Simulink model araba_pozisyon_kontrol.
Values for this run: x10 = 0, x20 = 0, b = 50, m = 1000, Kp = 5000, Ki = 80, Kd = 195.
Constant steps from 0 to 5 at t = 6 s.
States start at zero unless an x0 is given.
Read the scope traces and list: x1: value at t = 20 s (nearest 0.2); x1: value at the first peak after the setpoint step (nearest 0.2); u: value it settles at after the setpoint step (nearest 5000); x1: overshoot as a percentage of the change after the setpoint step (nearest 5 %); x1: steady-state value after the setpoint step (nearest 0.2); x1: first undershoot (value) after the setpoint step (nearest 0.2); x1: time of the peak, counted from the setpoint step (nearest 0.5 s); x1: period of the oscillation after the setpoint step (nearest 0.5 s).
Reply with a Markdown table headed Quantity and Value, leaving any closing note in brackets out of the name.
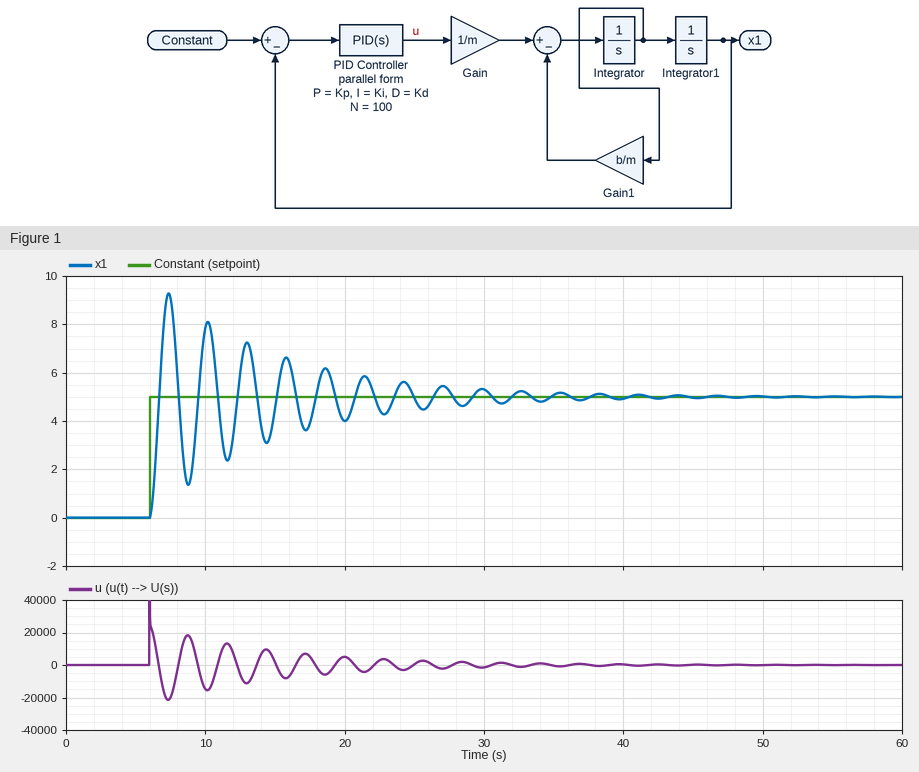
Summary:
| Quantity | Value |
|---|---|
| x1: value at t = 20 s | 4.0 |
| x1: value at the first peak after the setpoint step | 9.2 |
| u: value it settles at after the setpoint step | 0 |
| x1: overshoot as a percentage of the change after the setpoint step | 85 % |
| x1: steady-state value after the setpoint step | 5.0 |
| x1: first undershoot (value) after the setpoint step | 1.4 |
| x1: time of the peak, counted from the setpoint step | 1.5 s |
| x1: period of the oscillation after the setpoint step | 3.0 s |
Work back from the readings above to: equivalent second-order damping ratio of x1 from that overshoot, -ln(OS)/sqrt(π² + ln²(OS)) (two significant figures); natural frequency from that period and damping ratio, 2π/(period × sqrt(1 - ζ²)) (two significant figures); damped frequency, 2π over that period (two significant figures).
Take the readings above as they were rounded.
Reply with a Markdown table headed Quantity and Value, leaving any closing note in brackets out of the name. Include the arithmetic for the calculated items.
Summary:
| Quantity | Value |
|---|---|
| equivalent second-order damping ratio of x1 from that overshoot, -ln(OS)/sqrt(π² + ln²(OS)) | ln(0.85) = -0.163; 0.163 / sqrt(9.870 + 0.026) = 0.052 |
| natural frequency from that period and damping ratio, 2π/(period × sqrt(1 - ζ²)) | 2π / (3 × sqrt(1 - 0.052²)) = 2.1 rad/s |
| damped frequency, 2π over that period | 2π / 3 = 2.1 rad/s |
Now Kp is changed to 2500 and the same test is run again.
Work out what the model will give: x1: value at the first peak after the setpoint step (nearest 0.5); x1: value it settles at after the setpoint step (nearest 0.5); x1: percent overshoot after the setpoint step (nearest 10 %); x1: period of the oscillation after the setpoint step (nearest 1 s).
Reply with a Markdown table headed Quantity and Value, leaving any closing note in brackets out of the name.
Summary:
| Quantity | Value |
|---|---|
| x1: value at the first peak after the setpoint step | 9.0 |
| x1: value it settles at after the setpoint step | 5.0 |
| x1: percent overshoot after the setpoint step | 80 % |
| x1: period of the oscillation after the setpoint step | 4 s |
